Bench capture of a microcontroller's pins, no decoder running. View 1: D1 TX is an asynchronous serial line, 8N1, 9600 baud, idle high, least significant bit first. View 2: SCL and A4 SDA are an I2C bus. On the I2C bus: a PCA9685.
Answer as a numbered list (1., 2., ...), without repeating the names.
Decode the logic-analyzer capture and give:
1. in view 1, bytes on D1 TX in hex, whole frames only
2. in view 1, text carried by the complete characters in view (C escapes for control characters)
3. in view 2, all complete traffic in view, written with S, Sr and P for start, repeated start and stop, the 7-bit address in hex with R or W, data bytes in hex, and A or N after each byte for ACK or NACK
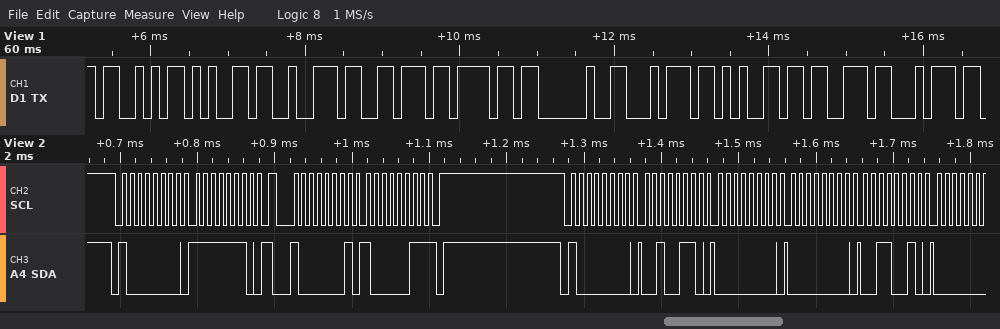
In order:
1. 53 65 72 76 6F 20 74 65 73 74
2. "Servo test"
3. S 40W A FE A Sr 40R A 83 N P S 40W A 26 A 00 A 00 A 32 A
